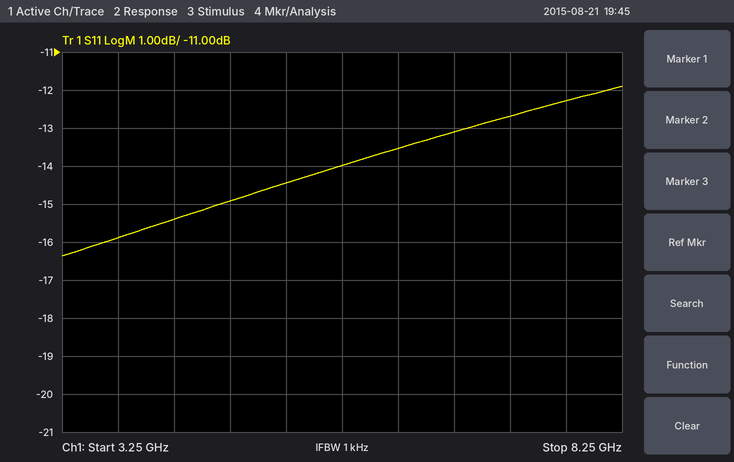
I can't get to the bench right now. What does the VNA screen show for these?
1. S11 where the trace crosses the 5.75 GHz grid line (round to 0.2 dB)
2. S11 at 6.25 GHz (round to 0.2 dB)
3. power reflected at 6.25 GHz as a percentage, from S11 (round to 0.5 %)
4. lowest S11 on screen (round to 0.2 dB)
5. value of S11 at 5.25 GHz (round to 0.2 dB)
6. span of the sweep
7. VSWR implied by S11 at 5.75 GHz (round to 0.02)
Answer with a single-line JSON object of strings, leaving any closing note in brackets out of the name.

{"S11 where the trace crosses the 5.75 GHz grid line": "-14.0 dB", "S11 at 6.25 GHz": "-13.6 dB", "power reflected at 6.25 GHz as a percentage, from S11": "4.5 %", "lowest S11 on screen": "-16.4 dB", "value of S11 at 5.25 GHz": "-14.4 dB", "span of the sweep": "5 GHz", "VSWR implied by S11 at 5.75 GHz": "1.50"}
